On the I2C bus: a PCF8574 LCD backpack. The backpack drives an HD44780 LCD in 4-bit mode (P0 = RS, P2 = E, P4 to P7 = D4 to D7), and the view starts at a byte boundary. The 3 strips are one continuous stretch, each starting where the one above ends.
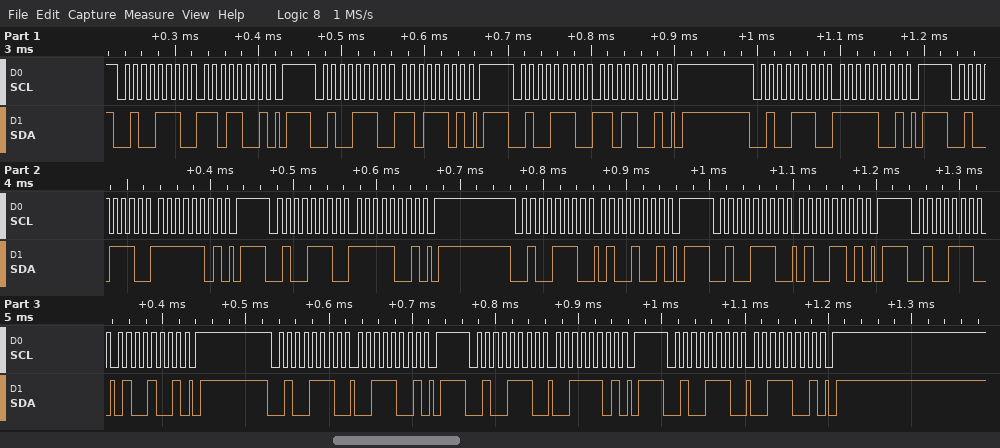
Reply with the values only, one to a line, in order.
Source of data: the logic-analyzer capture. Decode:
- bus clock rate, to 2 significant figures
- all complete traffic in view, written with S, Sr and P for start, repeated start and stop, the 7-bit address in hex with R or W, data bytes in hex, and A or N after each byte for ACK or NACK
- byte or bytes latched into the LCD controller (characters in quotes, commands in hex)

100 kHz
S 27W A D9 A P S 27W A DD A P S 27W A D9 A P S 27W A F9 A P S 27W A FD A P S 27W A F9 A P S 27W A 49 A P S 27W A 4D A P S 27W A 49 A P S 27W A 39 A P S 27W A 3D A P S 27W A 39 A P
data 0xDF 'C'
